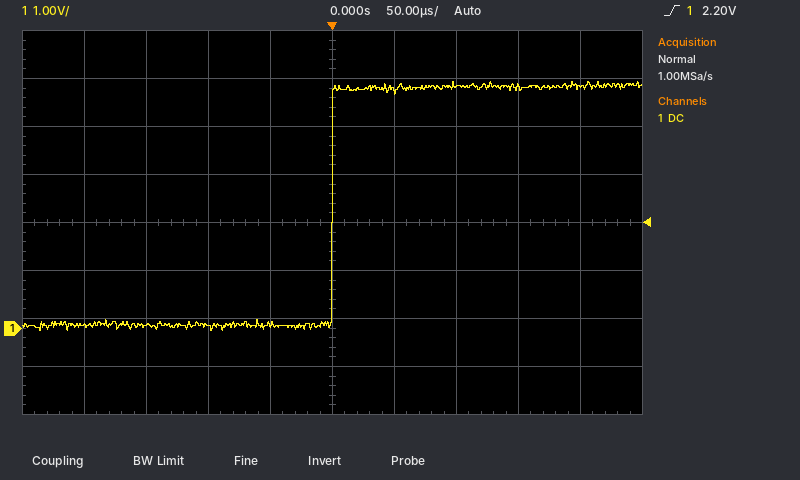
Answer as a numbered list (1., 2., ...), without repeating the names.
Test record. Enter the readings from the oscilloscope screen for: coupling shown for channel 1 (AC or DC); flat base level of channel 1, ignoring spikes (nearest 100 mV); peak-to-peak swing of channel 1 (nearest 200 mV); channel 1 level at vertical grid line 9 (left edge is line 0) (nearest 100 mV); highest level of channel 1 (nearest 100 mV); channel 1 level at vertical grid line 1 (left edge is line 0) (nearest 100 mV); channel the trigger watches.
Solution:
1. DC
2. 100 mV
3. 5.2 V
4. 5.0 V
5. 5.1 V
6. 100 mV
7. channel 1
